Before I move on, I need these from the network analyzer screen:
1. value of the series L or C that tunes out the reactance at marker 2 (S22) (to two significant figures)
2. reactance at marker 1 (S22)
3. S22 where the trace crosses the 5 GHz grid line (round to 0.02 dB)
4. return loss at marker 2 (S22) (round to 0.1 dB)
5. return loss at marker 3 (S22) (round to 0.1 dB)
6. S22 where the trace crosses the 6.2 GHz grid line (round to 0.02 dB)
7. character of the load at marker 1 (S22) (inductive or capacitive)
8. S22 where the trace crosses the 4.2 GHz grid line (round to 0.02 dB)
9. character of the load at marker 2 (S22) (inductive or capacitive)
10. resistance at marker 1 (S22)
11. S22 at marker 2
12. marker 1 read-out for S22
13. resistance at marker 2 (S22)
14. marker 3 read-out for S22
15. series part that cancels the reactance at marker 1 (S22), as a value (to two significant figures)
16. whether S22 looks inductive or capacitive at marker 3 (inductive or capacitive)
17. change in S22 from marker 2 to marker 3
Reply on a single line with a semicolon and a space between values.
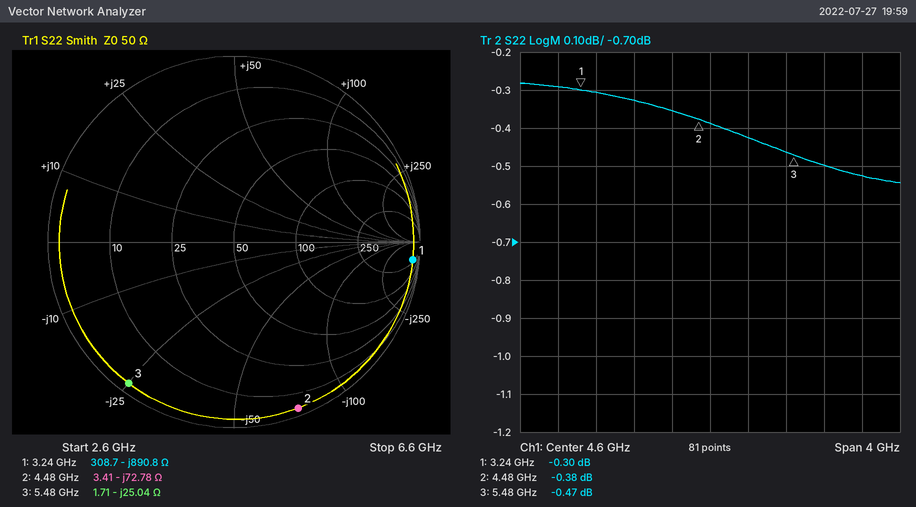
2.6 nH; -890.8 Ω; -0.42 dB; 0.4 dB; 0.5 dB; -0.52 dB; capacitive; -0.36 dB; capacitive; 308.7 Ω; -0.38 dB; -0.30 dB; 3.41 Ω; -0.47 dB; 44 nH; capacitive; -0.09 dB
